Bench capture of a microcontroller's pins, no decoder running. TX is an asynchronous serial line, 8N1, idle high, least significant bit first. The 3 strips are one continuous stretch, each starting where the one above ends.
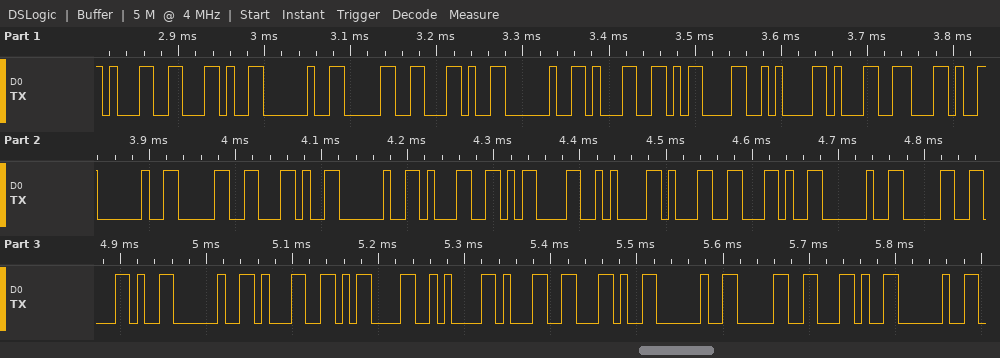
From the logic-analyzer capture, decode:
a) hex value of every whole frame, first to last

31 2C 20 30 2C 20 31 0D 0A 31 2C 20 30 2C 20 31 0D 0A 31 2C 20 30 2C 20 31 0D 0A 31 2C 20 30 2C 20
